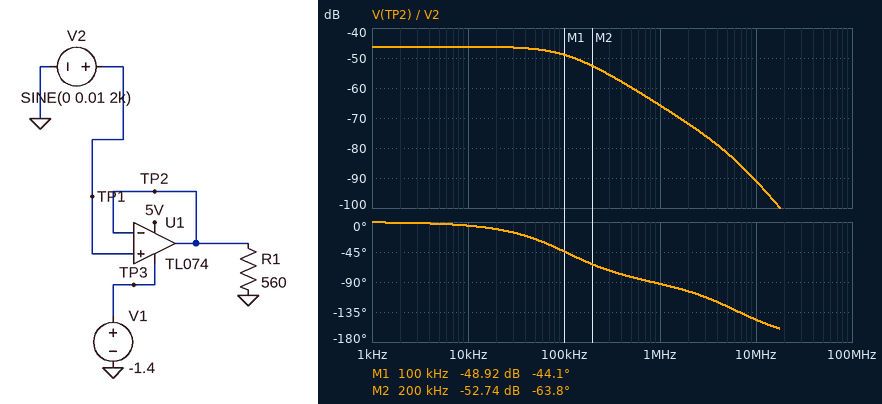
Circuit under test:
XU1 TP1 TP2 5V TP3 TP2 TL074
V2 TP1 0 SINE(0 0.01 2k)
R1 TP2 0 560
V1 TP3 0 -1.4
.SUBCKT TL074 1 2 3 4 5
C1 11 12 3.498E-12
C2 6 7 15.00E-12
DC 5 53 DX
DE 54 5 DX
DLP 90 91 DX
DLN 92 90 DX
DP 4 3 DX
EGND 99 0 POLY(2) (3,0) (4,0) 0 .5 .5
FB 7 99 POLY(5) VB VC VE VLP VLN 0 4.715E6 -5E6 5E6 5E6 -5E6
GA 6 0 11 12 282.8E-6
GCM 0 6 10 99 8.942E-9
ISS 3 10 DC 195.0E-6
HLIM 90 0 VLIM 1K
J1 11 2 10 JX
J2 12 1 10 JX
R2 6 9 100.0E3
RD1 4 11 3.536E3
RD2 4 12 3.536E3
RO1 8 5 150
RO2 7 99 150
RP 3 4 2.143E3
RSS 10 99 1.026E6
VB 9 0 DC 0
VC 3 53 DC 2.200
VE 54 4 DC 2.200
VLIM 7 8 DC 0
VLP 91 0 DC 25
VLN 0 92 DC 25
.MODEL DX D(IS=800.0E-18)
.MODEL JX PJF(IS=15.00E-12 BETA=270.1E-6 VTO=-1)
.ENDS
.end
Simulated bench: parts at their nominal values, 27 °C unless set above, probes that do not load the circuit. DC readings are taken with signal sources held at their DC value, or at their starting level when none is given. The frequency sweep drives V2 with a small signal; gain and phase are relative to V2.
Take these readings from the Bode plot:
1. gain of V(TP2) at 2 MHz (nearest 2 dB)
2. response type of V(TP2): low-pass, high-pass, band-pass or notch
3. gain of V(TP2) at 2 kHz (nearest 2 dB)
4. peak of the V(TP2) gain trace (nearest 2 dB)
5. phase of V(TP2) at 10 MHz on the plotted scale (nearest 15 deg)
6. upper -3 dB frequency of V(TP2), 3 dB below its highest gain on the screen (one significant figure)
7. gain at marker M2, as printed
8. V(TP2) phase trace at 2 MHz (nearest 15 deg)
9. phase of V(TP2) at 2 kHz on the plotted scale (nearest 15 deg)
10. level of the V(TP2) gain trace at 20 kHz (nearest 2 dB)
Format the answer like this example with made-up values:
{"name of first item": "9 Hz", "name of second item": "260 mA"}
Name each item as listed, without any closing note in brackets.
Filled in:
{"gain of V(TP2) at 2 MHz": "-72 dB", "response type of V(TP2): low-pass, high-pass, band-pass or notch": "low-pass", "gain of V(TP2) at 2 kHz": "-46 dB", "peak of the V(TP2) gain trace": "-46 dB", "phase of V(TP2) at 10 MHz on the plotted scale": "-150 deg", "upper -3 dB frequency of V(TP2), 3 dB below its highest gain on the screen": "100 kHz", "gain at marker M2, as printed": "-52.74 dB", "V(TP2) phase trace at 2 MHz": "-105 deg", "phase of V(TP2) at 2 kHz on the plotted scale": "0 deg", "level of the V(TP2) gain trace at 20 kHz": "-46 dB"}
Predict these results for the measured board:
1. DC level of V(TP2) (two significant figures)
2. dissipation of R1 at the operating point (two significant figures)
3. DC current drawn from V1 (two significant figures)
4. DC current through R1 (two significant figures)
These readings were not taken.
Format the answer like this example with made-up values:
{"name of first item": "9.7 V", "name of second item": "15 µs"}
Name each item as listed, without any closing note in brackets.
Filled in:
{"DC level of V(TP2)": "68 mV", "dissipation of R1 at the operating point": "8.2 µW", "DC current drawn from V1": "20 µA", "DC current through R1": "120 µA"}
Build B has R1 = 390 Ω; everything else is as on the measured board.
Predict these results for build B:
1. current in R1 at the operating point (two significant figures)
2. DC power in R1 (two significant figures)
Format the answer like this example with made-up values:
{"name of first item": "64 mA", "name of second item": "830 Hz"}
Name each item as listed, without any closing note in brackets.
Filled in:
{"current in R1 at the operating point": "170 µA", "DC power in R1": "12 µW"}
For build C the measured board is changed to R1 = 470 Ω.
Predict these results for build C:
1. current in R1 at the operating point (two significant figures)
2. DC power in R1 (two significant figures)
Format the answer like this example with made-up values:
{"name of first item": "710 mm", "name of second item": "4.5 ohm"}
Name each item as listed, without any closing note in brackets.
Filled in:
{"current in R1 at the operating point": "140 µA", "DC power in R1": "9.7 µW"}
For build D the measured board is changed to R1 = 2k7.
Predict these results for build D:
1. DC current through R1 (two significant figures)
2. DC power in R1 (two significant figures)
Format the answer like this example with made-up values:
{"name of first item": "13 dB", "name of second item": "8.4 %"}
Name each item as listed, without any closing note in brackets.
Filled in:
{"DC current through R1": "25 µA", "DC power in R1": "1.7 µW"}
